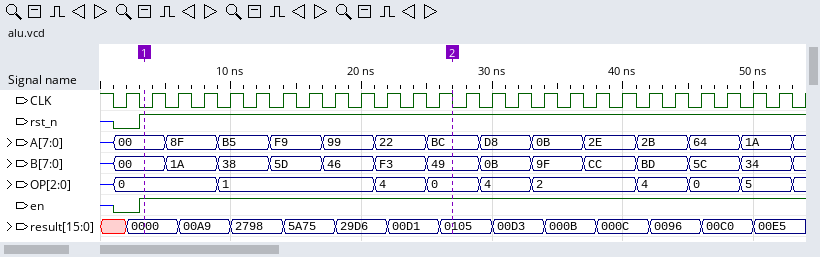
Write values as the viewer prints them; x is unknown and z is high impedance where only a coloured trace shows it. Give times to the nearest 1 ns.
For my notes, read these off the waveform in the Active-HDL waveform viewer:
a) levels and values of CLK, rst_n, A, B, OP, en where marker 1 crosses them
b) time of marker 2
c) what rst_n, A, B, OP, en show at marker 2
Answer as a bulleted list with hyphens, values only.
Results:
- CLK=0, rst_n=1, A=00, B=00, OP=0, en=1
- 27 ns
- rst_n=1, A=BC, B=49, OP=0, en=1
